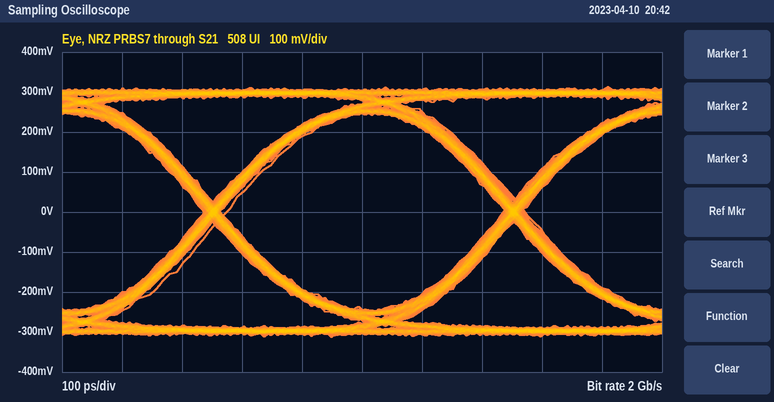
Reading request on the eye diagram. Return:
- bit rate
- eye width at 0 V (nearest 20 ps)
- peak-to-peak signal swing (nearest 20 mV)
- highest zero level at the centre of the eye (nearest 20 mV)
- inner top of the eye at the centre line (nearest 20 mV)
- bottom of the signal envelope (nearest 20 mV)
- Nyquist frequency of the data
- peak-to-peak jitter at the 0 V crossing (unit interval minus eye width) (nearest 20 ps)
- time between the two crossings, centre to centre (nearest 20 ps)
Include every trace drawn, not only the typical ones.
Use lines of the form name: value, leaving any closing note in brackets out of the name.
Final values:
bit rate: 2 Gb/s
eye width at 0 V: 460 ps
peak-to-peak signal swing: 620 mV
highest zero level at the centre of the eye: -240 mV
inner top of the eye at the centre line: 240 mV
bottom of the signal envelope: -320 mV
Nyquist frequency of the data: 1 GHz
peak-to-peak jitter at the 0 V crossing (unit interval minus eye width): 40 ps
time between the two crossings, centre to centre: 500 ps
